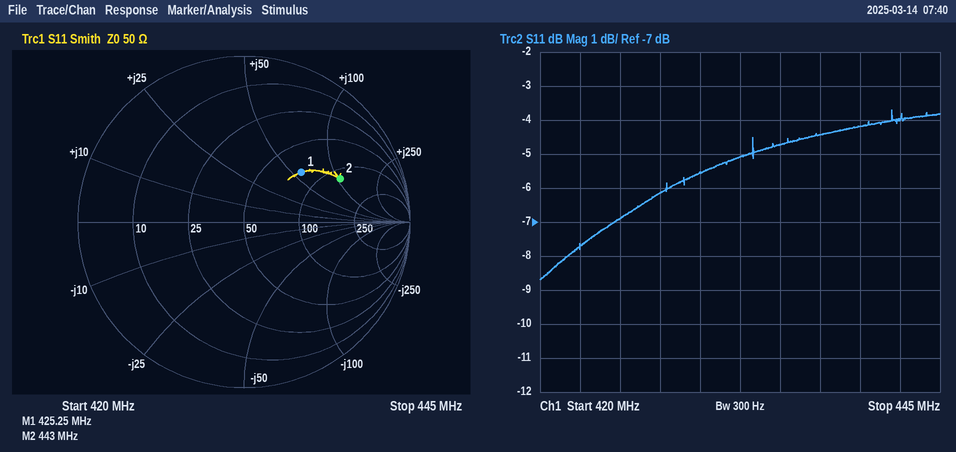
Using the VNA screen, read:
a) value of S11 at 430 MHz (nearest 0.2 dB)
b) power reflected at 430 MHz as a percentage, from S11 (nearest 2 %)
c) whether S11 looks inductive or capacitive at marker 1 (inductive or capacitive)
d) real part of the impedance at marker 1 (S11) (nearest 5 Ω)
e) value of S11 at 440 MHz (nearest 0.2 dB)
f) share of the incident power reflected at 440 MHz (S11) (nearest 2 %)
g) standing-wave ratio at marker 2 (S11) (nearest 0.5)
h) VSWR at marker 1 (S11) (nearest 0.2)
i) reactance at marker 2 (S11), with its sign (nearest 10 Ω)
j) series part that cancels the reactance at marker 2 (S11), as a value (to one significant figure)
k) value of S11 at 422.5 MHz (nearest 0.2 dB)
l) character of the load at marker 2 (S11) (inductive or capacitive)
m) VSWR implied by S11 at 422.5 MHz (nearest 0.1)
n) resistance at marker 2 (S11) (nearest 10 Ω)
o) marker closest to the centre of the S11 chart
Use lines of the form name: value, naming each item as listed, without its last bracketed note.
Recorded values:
value of S11 at 430 MHz: -5.6 dB
power reflected at 430 MHz as a percentage, from S11: 28 %
whether S11 looks inductive or capacitive at marker 1: inductive
real part of the impedance at marker 1 (S11): 75 Ω
value of S11 at 440 MHz: -4.2 dB
share of the incident power reflected at 440 MHz (S11): 38 %
standing-wave ratio at marker 2 (S11): 4.5
VSWR at marker 1 (S11): 2.6
reactance at marker 2 (S11), with its sign: +110 Ω
series part that cancels the reactance at marker 2 (S11), as a value: 3 pF
value of S11 at 422.5 MHz: -7.6 dB
character of the load at marker 2 (S11): inductive
VSWR implied by S11 at 422.5 MHz: 2.4
resistance at marker 2 (S11): 120 Ω
marker closest to the centre of the S11 chart: marker 1
